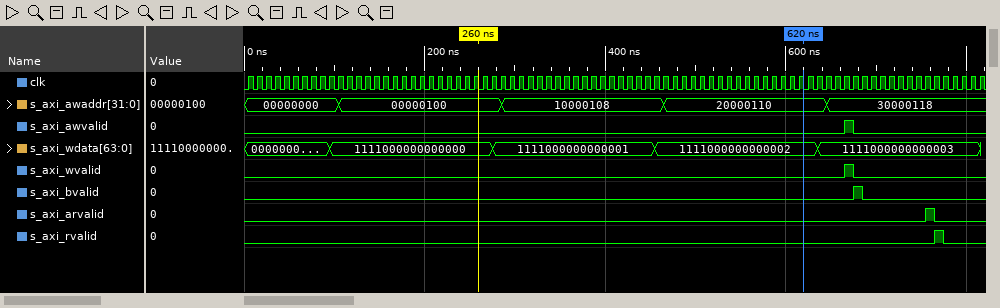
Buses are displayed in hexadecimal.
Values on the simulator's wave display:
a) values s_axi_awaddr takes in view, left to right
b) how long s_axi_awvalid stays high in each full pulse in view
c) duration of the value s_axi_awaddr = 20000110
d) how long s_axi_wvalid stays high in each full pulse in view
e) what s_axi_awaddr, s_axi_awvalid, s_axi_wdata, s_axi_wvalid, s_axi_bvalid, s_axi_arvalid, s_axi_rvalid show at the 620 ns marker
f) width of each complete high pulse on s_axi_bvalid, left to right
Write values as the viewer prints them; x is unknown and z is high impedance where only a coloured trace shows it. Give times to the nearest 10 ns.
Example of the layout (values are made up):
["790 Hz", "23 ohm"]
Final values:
["00000000, 00000100, 10000108, 20000110, 30000118", "10 ns", "180 ns", "10 ns", "s_axi_awaddr=20000110, s_axi_awvalid=0, s_axi_wdata=1111000000000002, s_axi_wvalid=0, s_axi_bvalid=0, s_axi_arvalid=0, s_axi_rvalid=0", "10 ns"]
